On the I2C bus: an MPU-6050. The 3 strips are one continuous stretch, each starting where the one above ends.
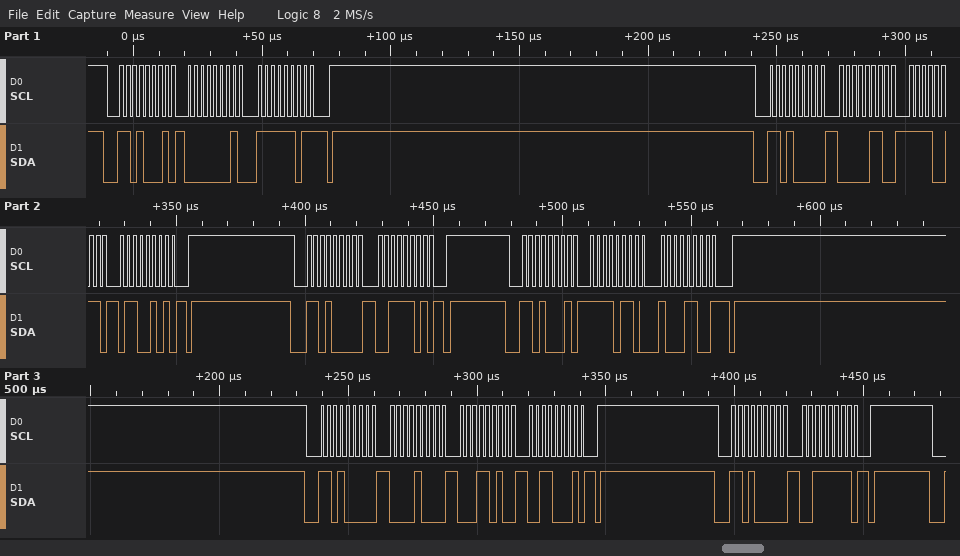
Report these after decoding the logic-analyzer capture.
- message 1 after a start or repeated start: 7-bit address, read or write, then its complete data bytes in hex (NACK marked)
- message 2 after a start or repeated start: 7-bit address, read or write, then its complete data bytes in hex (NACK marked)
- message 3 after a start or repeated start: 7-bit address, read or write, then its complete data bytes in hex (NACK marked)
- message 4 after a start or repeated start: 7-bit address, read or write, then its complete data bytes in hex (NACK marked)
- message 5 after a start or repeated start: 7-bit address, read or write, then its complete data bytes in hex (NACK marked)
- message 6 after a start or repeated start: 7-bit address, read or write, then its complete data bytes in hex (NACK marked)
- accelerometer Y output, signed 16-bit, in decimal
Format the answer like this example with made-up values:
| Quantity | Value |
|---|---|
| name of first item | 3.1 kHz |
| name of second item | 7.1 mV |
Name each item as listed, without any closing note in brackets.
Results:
| Quantity | Value |
|---|---|
| message 1 after a start or repeated start: 7-bit address, read or write, then its complete data bytes in hex | 0x68 read: 01 FD NACK |
| message 2 after a start or repeated start: 7-bit address, read or write, then its complete data bytes in hex | 0x68 write: 06 F3 65 |
| message 3 after a start or repeated start: 7-bit address, read or write, then its complete data bytes in hex | 0x68 write: 3D |
| message 4 after a start or repeated start: 7-bit address, read or write, then its complete data bytes in hex | 0x68 read: F6 8C NACK |
| message 5 after a start or repeated start: 7-bit address, read or write, then its complete data bytes in hex | 0x68 write: 08 1A 31 |
| message 6 after a start or repeated start: 7-bit address, read or write, then its complete data bytes in hex | 0x68 write: 3F |
| accelerometer Y output, signed 16-bit, in decimal | -2420 |
